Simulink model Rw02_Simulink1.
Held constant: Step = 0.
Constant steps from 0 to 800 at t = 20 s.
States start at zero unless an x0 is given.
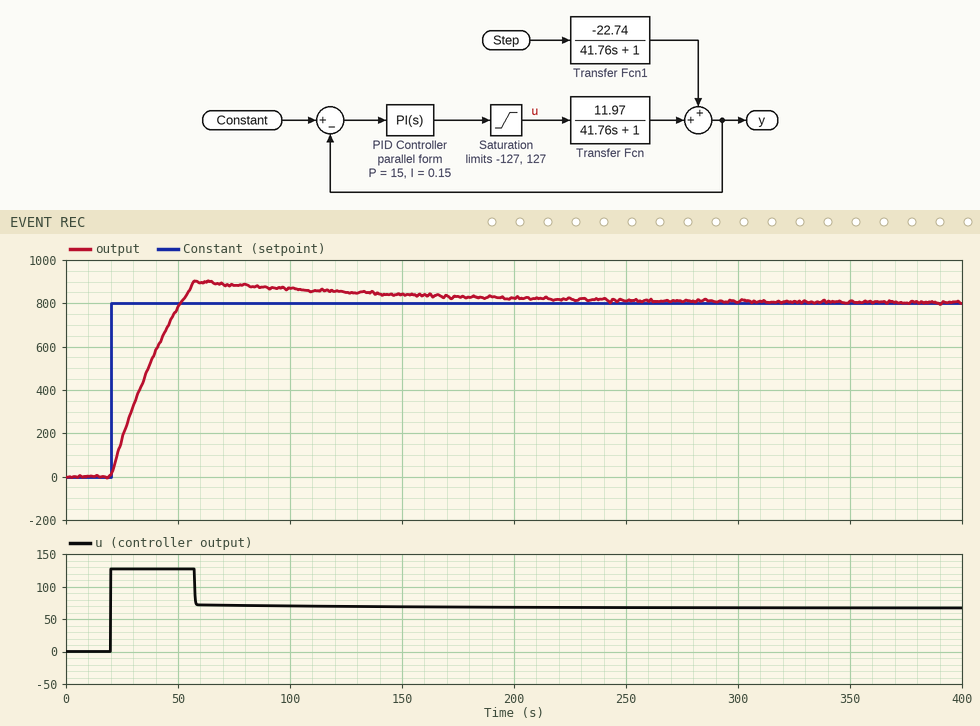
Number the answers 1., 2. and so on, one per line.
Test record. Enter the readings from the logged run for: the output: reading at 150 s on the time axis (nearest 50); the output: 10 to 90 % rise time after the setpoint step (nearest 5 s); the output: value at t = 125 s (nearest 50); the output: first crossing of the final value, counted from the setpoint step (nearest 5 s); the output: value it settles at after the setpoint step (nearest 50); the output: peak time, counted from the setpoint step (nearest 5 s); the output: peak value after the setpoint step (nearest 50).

1. 850
2. 25 s
3. 850
4. 30 s
5. 800
6. 40 s
7. 900
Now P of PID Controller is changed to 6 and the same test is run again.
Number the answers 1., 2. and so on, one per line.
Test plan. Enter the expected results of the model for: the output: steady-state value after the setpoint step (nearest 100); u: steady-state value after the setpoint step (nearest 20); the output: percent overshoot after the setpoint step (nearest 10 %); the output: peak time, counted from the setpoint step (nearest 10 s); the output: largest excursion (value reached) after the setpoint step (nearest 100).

1. 800
2. 60
3. 30 %
4. 50 s
5. 1000
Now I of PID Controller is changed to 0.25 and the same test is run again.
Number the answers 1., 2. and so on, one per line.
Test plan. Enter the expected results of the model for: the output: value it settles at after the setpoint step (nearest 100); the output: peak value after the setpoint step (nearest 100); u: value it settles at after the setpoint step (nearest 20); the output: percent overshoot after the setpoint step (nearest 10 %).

1. 800
2. 1000
3. 60
4. 20 %
